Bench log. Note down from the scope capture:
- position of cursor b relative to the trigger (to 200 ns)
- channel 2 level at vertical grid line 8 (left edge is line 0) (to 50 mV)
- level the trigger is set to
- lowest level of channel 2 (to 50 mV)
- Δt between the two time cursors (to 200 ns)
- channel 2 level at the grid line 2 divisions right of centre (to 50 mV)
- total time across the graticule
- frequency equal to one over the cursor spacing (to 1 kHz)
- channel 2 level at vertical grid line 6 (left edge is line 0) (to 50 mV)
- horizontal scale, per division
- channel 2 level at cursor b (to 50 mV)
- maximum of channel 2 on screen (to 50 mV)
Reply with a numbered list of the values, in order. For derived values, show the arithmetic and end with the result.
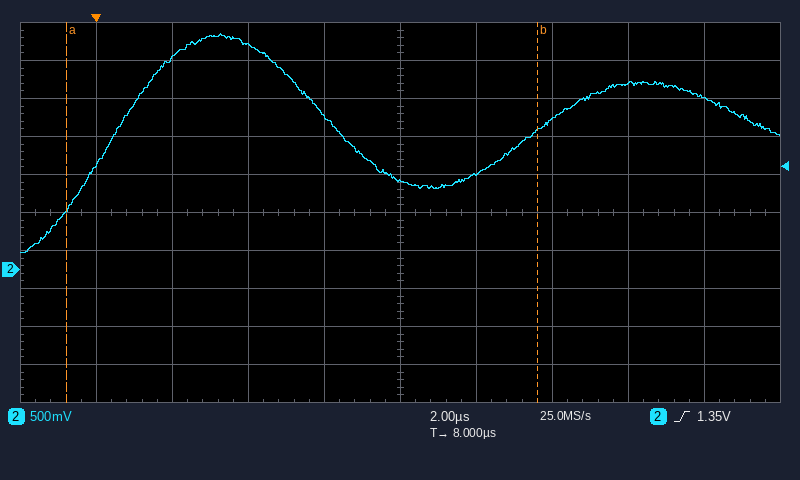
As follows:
1. +11.6 µs
2. 2.45 V
3. 1.35 V
4. 200 mV
5. 12.4 µs
6. 2.00 V
7. 20 µs
8. 1 / 12.4 µs ≈ 81 kHz
9. 1.25 V
10. 2 µs
11. 1.85 V
12. 3.10 V
